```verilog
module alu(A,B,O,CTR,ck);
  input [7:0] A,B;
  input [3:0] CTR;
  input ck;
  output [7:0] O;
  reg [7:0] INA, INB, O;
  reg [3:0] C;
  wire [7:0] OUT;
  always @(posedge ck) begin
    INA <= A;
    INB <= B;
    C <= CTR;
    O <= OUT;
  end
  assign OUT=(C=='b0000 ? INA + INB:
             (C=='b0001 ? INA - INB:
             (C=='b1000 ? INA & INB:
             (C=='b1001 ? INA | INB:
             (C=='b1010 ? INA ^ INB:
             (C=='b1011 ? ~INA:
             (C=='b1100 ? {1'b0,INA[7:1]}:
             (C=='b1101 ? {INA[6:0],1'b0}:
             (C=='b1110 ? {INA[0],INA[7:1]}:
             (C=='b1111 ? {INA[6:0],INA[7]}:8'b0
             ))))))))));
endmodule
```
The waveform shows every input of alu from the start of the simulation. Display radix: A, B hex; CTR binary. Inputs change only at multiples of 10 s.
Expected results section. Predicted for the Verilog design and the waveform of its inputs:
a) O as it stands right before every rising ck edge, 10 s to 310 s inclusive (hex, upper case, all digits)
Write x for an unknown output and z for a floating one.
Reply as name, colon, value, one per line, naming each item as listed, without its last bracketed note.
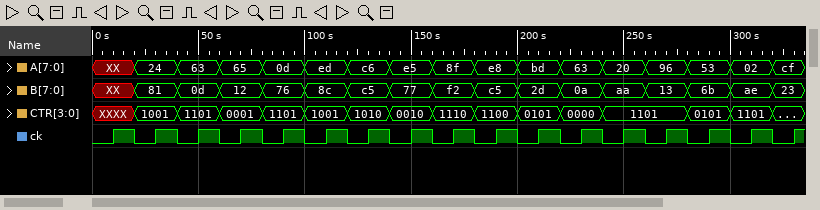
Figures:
O as it stands right before every rising ck edge, 10 s to 310 s inclusive: x, x, x, A5, C6, 53, 1A, ED, 03, 00, C7, 74, 00, 6D, 40, 2C
